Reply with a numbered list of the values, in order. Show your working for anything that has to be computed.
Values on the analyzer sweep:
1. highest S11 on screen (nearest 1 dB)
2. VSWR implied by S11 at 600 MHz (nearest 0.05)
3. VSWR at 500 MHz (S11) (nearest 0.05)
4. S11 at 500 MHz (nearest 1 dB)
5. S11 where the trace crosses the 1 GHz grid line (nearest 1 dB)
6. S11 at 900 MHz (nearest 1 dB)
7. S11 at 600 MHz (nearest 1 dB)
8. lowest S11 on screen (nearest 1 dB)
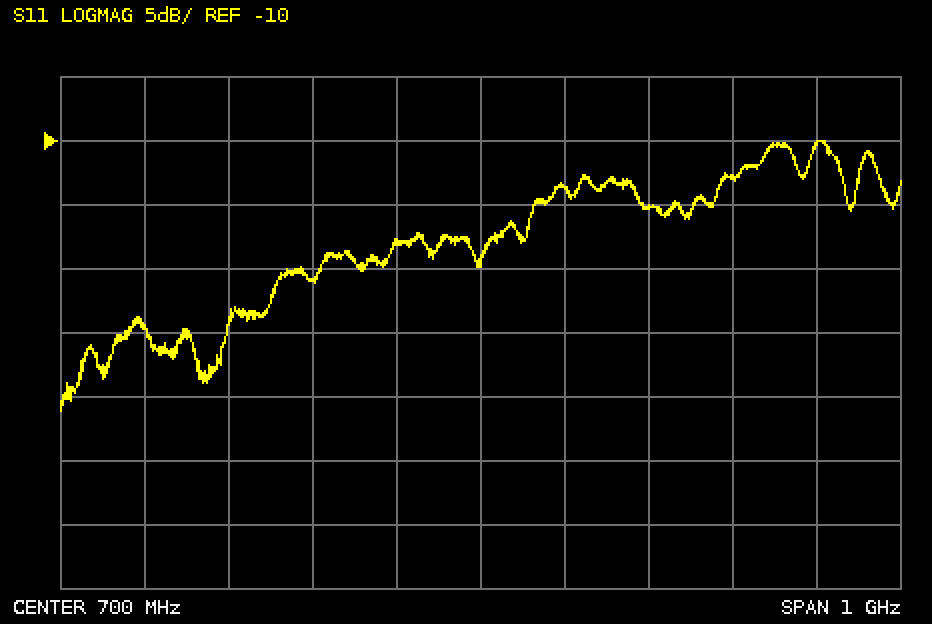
1. -10 dB
2. |Γ| = 10^(-18/20) = 0.1259; VSWR = (1 + 0.1259)/(1 − 0.1259) ≈ 1.29, so 1.30 to the nearest 0.05
3. |Γ| = 10^(-21/20) = 0.0891; VSWR = (1 + 0.0891)/(1 − 0.0891) ≈ 1.20
4. -21 dB
5. -13 dB
6. -15 dB
7. -18 dB
8. -31 dB
